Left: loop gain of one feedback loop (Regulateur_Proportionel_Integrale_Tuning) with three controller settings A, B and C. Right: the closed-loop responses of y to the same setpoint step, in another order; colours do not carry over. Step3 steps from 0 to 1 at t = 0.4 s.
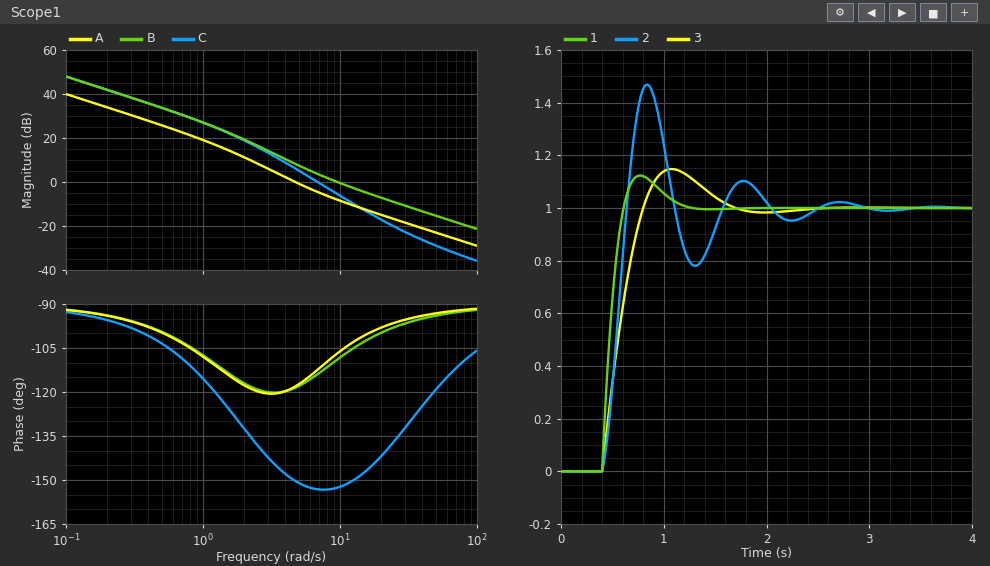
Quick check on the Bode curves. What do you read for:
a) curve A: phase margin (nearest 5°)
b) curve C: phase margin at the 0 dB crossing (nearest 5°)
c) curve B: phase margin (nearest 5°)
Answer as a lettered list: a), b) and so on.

a) 60°
b) 25°
c) 70°
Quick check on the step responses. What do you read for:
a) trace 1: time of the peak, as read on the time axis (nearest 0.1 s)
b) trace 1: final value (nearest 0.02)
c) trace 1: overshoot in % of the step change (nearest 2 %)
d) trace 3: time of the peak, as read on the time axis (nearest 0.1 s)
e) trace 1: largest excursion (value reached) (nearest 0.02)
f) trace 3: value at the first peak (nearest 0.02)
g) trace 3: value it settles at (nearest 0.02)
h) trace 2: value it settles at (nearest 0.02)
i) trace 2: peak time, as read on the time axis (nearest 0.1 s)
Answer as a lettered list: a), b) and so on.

a) 0.8 s
b) 1.00
c) 12 %
d) 1.1 s
e) 1.12
f) 1.14
g) 1.00
h) 1.00
i) 0.8 s
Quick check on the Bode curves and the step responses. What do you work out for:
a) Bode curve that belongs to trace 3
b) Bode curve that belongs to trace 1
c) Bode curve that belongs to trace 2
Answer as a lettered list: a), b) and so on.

a) A
b) B
c) C
